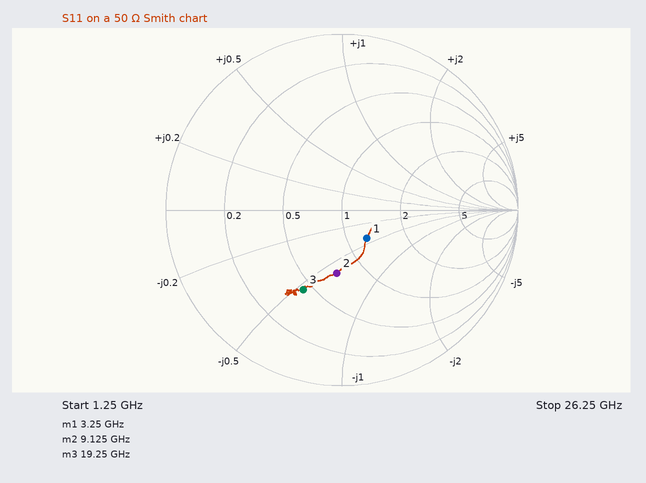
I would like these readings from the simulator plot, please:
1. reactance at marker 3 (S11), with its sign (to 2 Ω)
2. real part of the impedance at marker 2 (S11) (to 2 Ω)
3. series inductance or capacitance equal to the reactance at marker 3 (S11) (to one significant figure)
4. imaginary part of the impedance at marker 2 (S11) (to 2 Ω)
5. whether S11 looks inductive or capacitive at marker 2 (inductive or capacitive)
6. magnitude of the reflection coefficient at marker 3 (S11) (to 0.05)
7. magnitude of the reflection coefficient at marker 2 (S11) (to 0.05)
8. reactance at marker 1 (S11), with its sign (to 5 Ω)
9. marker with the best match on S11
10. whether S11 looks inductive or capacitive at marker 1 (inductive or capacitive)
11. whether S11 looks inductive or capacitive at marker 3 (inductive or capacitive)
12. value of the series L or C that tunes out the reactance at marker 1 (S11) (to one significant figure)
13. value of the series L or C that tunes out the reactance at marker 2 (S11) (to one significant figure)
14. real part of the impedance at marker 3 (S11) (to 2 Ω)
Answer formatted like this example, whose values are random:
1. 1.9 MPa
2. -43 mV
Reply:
1. -26 Ω
2. 36 Ω
3. 300 fF
4. -30 Ω
5. capacitive
6. 0.50
7. 0.35
8. -20 Ω
9. marker 1
10. capacitive
11. capacitive
12. 1 nH
13. 500 pH
14. 22 Ω
